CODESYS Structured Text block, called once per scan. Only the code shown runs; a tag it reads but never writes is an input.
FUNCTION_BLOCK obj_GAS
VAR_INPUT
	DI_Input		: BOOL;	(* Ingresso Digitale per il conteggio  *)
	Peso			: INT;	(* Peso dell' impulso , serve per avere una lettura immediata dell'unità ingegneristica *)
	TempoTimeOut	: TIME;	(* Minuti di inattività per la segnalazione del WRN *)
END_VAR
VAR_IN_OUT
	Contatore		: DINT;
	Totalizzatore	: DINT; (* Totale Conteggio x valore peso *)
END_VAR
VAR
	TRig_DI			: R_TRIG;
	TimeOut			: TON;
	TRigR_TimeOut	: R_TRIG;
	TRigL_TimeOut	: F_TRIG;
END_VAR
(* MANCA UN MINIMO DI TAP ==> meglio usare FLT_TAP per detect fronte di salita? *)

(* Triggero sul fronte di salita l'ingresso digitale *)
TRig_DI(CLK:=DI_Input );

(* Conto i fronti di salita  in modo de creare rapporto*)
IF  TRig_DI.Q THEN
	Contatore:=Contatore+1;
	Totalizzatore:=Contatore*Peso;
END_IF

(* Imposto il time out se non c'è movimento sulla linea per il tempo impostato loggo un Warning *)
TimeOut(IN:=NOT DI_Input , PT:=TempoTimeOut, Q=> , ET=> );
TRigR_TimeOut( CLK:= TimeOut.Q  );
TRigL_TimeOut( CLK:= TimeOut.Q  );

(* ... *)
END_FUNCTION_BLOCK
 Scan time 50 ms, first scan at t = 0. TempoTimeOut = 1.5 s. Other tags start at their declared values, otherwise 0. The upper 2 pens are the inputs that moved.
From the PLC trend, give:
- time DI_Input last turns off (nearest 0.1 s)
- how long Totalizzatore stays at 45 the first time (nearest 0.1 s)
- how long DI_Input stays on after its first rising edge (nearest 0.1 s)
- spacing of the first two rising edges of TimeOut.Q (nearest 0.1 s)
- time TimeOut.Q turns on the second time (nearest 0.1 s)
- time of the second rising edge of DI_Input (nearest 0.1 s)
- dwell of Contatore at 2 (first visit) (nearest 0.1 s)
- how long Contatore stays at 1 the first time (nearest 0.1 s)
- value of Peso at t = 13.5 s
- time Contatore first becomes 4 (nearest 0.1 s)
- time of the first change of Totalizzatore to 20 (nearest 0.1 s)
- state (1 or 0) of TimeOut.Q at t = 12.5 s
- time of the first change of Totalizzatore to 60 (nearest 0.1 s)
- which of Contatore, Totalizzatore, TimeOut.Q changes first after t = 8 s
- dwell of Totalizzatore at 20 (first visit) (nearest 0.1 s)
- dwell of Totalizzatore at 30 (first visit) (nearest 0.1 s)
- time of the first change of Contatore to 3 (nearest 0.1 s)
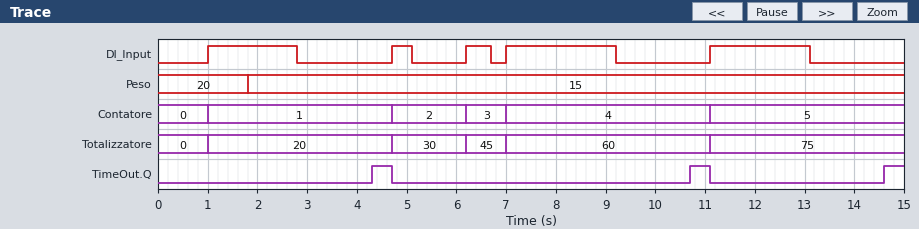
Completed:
13.1 s
0.8 s
1.8 s
6.4 s
10.7 s
4.7 s
1.5 s
3.7 s
15
7.0 s
1.0 s
0
7.0 s
TimeOut.Q
3.7 s
1.5 s
6.2 s
